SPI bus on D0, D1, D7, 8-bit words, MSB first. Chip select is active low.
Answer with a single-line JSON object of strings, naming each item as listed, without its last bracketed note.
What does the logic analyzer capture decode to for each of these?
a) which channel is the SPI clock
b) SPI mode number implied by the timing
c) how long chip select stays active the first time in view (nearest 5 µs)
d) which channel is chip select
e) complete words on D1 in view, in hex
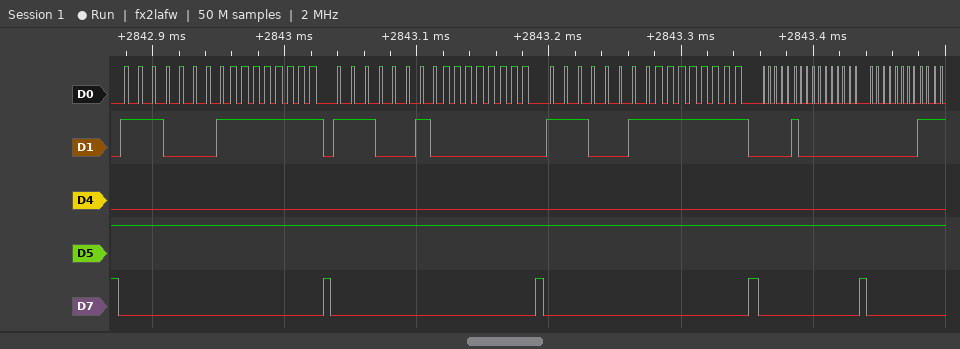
{"which channel is the SPI clock": "D0", "SPI mode number implied by the timing": "1", "how long chip select stays active the first time in view": "155 µs", "which channel is chip select": "D7", "complete words on D1 in view, in hex": "E1, FF, E2, 00, E3, FF, 04, 00, 00"}
